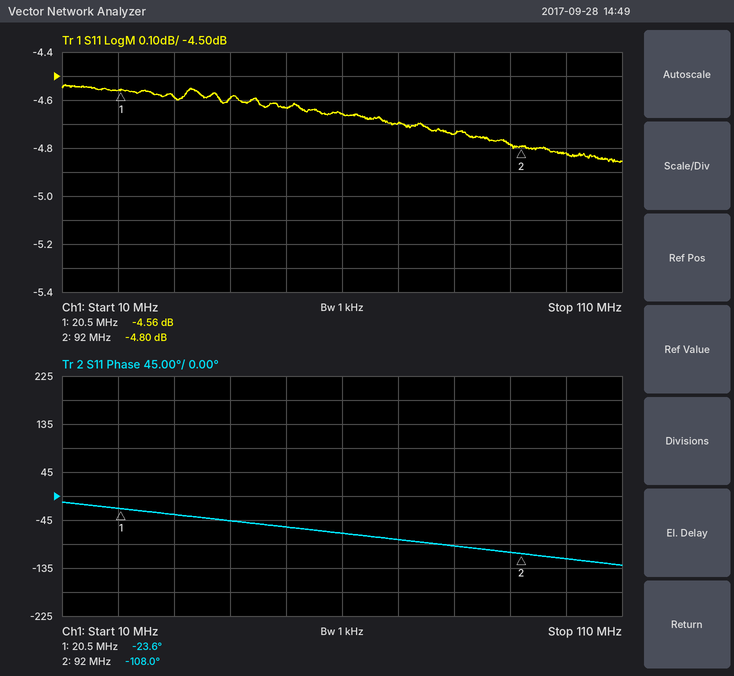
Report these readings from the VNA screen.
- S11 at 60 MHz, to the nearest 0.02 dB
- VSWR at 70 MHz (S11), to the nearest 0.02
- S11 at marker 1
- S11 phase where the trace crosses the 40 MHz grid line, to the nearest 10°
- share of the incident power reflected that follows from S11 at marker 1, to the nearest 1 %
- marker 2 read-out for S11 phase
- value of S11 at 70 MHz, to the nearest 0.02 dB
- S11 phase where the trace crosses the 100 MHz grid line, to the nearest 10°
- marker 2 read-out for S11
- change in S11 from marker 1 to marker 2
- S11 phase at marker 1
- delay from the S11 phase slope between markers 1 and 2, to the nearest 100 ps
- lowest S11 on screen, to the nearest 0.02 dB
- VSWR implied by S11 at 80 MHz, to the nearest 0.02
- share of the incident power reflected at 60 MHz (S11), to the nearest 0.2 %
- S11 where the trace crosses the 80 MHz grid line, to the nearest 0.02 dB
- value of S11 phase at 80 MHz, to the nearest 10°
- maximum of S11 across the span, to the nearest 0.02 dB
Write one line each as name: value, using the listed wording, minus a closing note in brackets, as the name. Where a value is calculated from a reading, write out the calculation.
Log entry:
S11 at 60 MHz, to the nearest 0.02 dB: -4.66 dB
VSWR at 70 MHz (S11), to the nearest 0.02: |Γ| = 10^(-4.7/20) = 0.5821; VSWR = (1 + 0.5821)/(1 − 0.5821) ≈ 3.79, so 3.78 to the nearest 0.02
S11 at marker 1: -4.56 dB
S11 phase where the trace crosses the 40 MHz grid line, to the nearest 10°: -50°
share of the incident power reflected that follows from S11 at marker 1, to the nearest 1 %: 10^(-4.56/10) ≈ 35 %
marker 2 read-out for S11 phase: -108.0°
value of S11 at 70 MHz, to the nearest 0.02 dB: -4.70 dB
S11 phase where the trace crosses the 100 MHz grid line, to the nearest 10°: -120°
marker 2 read-out for S11: -4.80 dB
change in S11 from marker 1 to marker 2: -4.8 − (-4.56) = -0.24 dB
S11 phase at marker 1: -23.6°
delay from the S11 phase slope between markers 1 and 2, to the nearest 100 ps: −(-108° − (-23.6°))/(360° × 71.5 MHz) ≈ 3.3 ns
lowest S11 on screen, to the nearest 0.02 dB: -4.86 dB
VSWR implied by S11 at 80 MHz, to the nearest 0.02: |Γ| = 10^(-4.74/20) = 0.5794; VSWR = (1 + 0.5794)/(1 − 0.5794) ≈ 3.76
share of the incident power reflected at 60 MHz (S11), to the nearest 0.2 %: 10^(-4.66/10) ≈ 34.2 %
S11 where the trace crosses the 80 MHz grid line, to the nearest 0.02 dB: -4.74 dB
value of S11 phase at 80 MHz, to the nearest 10°: -90°
maximum of S11 across the span, to the nearest 0.02 dB: -4.54 dB
